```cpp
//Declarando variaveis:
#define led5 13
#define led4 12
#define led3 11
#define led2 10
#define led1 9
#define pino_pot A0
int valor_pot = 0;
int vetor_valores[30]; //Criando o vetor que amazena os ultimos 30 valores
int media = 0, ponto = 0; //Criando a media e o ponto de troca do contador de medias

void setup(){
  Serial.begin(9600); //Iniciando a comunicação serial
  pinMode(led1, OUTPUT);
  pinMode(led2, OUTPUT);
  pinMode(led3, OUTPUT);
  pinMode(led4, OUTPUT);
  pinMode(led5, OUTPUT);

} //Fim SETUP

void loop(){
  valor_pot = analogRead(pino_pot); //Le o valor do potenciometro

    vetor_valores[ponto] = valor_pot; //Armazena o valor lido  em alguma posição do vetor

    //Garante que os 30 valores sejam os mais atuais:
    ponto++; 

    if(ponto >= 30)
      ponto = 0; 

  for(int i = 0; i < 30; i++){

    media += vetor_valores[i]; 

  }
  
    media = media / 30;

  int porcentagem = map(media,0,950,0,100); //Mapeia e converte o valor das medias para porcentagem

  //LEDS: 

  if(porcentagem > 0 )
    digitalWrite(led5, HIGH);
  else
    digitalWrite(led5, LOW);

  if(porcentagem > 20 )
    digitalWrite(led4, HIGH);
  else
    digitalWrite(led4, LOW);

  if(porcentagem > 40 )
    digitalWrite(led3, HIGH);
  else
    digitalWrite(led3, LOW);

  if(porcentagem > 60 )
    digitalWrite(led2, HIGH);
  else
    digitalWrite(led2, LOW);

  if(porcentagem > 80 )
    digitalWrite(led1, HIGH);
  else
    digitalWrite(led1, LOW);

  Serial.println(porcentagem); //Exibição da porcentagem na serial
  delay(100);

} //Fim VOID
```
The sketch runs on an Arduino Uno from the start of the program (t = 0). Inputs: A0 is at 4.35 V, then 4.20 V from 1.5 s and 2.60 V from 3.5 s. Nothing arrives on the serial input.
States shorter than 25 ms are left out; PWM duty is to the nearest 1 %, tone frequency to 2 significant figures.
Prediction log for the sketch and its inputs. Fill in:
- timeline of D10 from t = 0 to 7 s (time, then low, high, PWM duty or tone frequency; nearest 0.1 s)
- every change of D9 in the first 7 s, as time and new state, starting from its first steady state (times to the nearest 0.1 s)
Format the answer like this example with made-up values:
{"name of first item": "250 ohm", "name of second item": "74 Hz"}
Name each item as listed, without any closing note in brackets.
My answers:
{"timeline of D10 from t = 0 to 7 s": "0 s low; 1.9 s high; 6.2 s low", "every change of D9 in the first 7 s, as time and new state, starting from its first steady state": "0 s low; 2.5 s high; 4.5 s low"}
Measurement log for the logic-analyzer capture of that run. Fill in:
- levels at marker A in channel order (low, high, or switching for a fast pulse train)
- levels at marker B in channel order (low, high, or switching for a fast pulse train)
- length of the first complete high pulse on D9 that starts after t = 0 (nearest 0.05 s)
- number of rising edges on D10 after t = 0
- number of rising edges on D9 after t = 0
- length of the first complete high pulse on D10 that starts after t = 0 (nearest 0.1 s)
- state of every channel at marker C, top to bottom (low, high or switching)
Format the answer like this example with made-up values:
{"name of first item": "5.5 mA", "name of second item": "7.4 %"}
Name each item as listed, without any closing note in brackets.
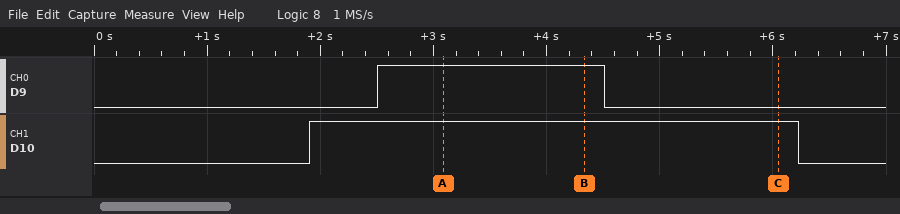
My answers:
{"levels at marker A in channel order": "D9 high, D10 high", "levels at marker B in channel order": "D9 high, D10 high", "length of the first complete high pulse on D9 that starts after t = 0": "2.00 s", "number of rising edges on D10 after t = 0": "1", "number of rising edges on D9 after t = 0": "1", "length of the first complete high pulse on D10 that starts after t = 0": "4.3 s", "state of every channel at marker C, top to bottom": "D9 low, D10 high"}
